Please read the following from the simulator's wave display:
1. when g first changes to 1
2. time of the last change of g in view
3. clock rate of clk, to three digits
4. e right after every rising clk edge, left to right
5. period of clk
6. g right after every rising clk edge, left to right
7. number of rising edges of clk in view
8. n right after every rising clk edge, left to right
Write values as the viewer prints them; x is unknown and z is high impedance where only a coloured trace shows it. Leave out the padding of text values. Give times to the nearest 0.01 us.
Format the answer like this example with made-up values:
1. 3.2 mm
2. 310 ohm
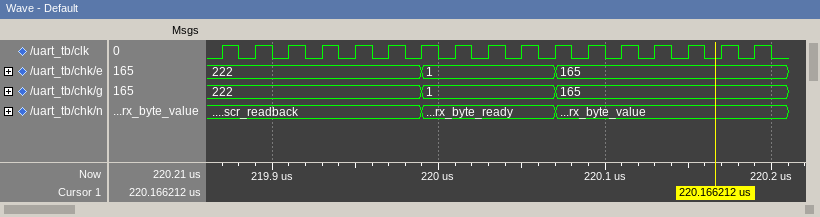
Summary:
1. 219.99 us
2. 220.07 us
3. 50.0 MHz
4. 222, 222, 222, 222, 222, 222, 1, 1, 1, 1, 165, 165, 165, 165, 165, 165, 165
5. 0.02 us
6. 222, 222, 222, 222, 222, 222, 1, 1, 1, 1, 165, 165, 165, 165, 165, 165, 165
7. 17
8. scr_readback, scr_readback, scr_readback, scr_readback, scr_readback, scr_readback, rx_byte_ready, rx_byte_ready, rx_byte_ready, rx_byte_ready, rx_byte_value, rx_byte_value, rx_byte_value, rx_byte_value, rx_byte_value, rx_byte_value, rx_byte_value
